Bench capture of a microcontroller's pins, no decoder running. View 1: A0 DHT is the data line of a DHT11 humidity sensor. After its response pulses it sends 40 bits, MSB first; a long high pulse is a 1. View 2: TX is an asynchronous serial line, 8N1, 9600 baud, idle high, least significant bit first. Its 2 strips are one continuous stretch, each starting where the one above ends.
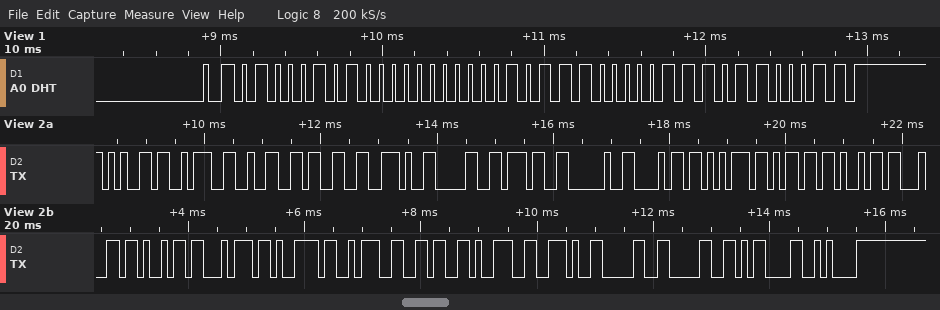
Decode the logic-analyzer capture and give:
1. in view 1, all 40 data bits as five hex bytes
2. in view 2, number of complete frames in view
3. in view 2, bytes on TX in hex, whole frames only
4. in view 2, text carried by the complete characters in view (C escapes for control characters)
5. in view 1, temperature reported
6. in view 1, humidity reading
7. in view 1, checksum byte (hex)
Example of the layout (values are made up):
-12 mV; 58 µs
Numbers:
45 00 17 07 63; 24; 65 3A 32 33 2E 30 37 20 68 75 6D 69 64 69 74 79 3A 36 39 2E 30 30 0D 0A; "e:23.07 humidity:69.00\r\n"; 23.7 °C; 69 %; 0x63
